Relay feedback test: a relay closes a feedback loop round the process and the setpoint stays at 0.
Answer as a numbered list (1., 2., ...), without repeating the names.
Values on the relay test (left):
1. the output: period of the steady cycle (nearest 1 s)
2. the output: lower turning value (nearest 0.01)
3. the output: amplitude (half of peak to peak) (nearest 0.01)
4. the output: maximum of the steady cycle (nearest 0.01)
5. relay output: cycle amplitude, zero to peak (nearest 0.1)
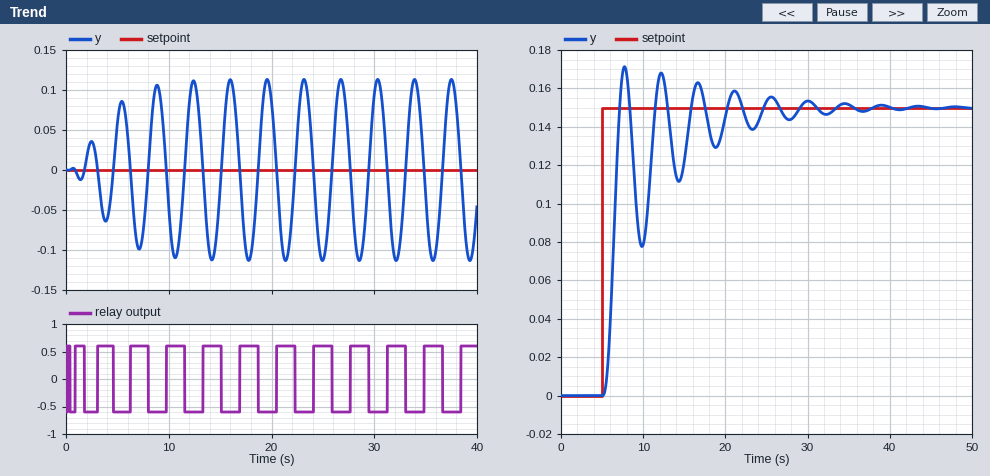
1. 4 s
2. -0.11
3. 0.11
4. 0.11
5. 0.6
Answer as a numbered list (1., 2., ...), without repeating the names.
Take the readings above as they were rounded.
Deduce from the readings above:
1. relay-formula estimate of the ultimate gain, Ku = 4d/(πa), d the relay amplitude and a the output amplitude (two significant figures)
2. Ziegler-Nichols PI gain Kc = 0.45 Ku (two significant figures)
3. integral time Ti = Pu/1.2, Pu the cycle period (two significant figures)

1. 6.9
2. 3.1
3. 3.3 s
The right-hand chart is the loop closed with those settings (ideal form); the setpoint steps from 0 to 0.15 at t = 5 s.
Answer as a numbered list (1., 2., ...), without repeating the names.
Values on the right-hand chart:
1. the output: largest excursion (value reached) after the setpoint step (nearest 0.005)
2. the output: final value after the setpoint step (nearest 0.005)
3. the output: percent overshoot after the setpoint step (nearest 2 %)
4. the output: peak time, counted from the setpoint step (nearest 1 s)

1. 0.170
2. 0.150
3. 14 %
4. 3 s
